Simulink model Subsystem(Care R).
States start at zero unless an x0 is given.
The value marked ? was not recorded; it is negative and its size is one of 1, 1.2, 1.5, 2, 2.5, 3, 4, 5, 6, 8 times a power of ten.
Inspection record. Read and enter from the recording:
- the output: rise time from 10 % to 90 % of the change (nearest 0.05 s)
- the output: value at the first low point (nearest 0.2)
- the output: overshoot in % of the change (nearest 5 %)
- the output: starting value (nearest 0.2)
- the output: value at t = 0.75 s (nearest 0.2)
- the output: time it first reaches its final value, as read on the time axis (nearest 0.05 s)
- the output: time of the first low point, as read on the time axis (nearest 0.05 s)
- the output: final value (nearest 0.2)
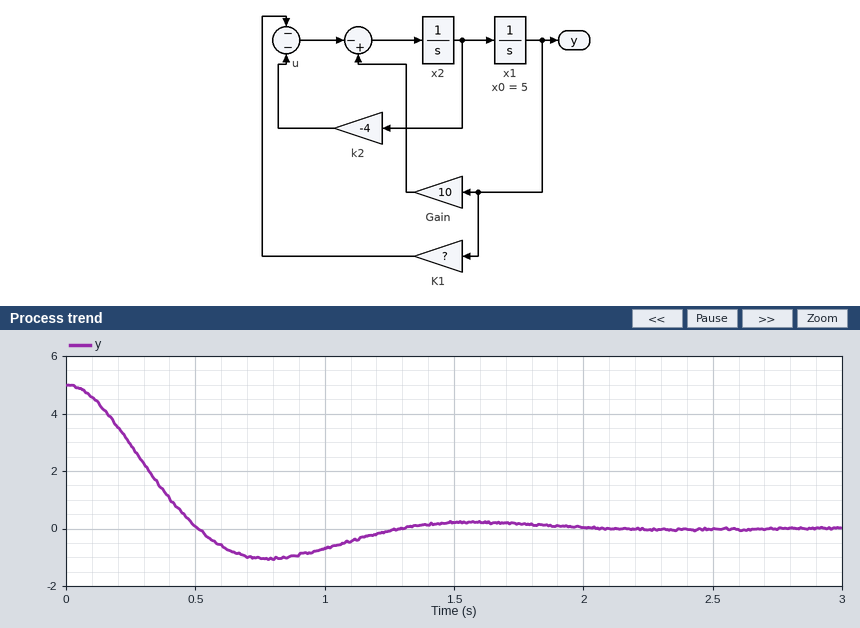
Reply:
0.35 s
-1.0
20 %
5.0
-1.0
0.50 s
0.80 s
0.0
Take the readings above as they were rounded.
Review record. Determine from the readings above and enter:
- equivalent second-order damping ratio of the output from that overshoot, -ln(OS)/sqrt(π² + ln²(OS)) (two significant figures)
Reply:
0.46
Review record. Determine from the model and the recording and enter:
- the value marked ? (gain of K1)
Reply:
-30
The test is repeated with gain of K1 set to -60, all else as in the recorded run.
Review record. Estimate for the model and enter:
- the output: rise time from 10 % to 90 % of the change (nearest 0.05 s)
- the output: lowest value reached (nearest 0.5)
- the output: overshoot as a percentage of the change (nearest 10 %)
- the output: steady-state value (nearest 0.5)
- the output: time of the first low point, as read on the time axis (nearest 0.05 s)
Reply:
0.20 s
-2.0
40 %
0.0
0.45 s
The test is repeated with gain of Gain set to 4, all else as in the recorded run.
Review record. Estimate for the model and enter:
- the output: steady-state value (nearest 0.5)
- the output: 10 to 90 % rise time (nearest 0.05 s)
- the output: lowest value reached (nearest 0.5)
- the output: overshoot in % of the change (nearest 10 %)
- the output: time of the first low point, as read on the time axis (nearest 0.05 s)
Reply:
0.0
0.30 s
-1.5
30 %
0.65 s
